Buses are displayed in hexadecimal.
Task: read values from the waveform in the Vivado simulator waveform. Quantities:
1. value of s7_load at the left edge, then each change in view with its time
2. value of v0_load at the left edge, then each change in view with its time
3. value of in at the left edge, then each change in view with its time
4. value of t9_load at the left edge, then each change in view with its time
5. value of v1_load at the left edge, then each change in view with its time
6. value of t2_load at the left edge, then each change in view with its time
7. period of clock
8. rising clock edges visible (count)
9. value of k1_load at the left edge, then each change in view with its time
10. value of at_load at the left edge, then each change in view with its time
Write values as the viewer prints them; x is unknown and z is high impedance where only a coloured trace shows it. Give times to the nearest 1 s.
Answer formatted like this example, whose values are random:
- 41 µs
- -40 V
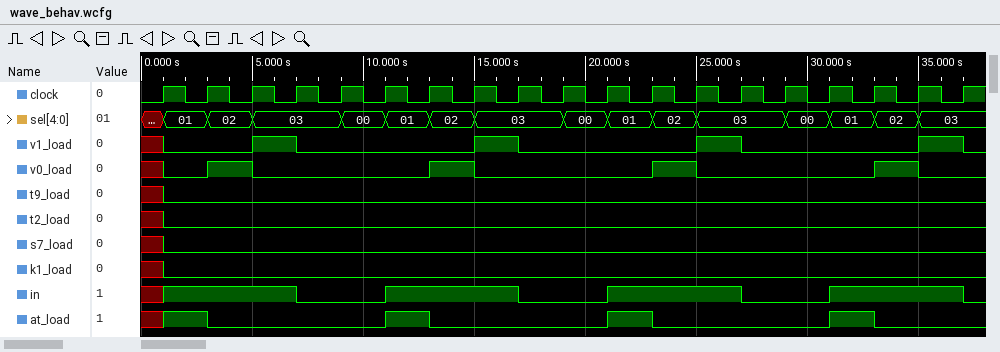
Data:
- x, 0 at 1 s
- x, 0 at 1 s, 1 at 3 s, 0 at 5 s, 1 at 13 s, 0 at 15 s, 1 at 23 s, 0 at 25 s, 1 at 33 s, 0 at 35 s
- x, 1 at 1 s, 0 at 7 s, 1 at 11 s, 0 at 17 s, 1 at 21 s, 0 at 27 s, 1 at 31 s, 0 at 37 s
- x, 0 at 1 s
- x, 0 at 1 s, 1 at 5 s, 0 at 7 s, 1 at 15 s, 0 at 17 s, 1 at 25 s, 0 at 27 s, 1 at 35 s, 0 at 37 s
- x, 0 at 1 s
- 2 s
- 19
- x, 0 at 1 s
- x, 1 at 1 s, 0 at 3 s, 1 at 11 s, 0 at 13 s, 1 at 21 s, 0 at 23 s, 1 at 31 s, 0 at 33 s
